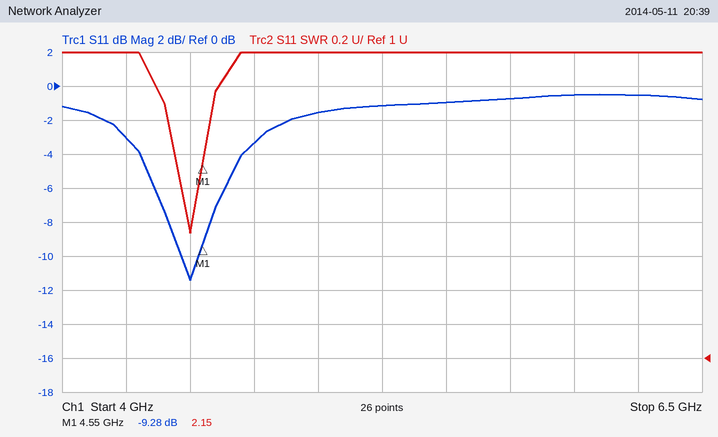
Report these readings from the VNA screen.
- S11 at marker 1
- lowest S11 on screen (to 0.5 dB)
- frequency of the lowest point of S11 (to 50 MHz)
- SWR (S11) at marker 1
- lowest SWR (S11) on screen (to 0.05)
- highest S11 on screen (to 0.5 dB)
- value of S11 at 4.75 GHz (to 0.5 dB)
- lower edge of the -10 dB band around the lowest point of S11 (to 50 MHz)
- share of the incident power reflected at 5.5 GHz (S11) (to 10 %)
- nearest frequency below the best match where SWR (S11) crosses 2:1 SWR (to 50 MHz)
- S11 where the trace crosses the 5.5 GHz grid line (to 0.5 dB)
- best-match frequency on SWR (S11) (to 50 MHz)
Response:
-9.28 dB
-11.5 dB
4.50 GHz
2.15
1.75
-0.5 dB
-3.5 dB
4.45 GHz
80 %
4.45 GHz
-1.0 dB
4.50 GHz
